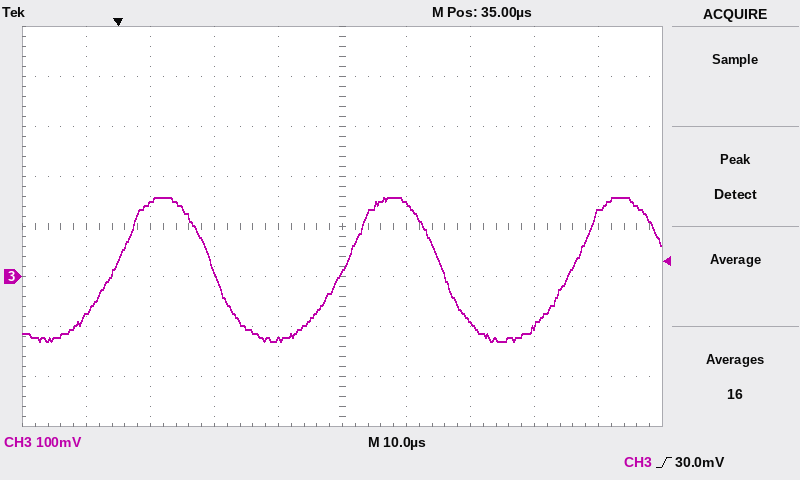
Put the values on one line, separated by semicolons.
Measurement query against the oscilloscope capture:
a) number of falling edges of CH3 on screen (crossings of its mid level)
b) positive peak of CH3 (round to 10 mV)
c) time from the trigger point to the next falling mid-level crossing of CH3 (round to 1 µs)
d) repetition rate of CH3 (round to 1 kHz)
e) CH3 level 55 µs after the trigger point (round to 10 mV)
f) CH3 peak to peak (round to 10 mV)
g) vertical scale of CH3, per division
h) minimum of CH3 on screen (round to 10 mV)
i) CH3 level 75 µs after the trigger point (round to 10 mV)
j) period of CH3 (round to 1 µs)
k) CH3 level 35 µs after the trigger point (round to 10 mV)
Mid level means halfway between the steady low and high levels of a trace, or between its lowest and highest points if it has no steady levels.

2; 160 mV; 15 µs; 28 kHz; -90 mV; 290 mV; 100 mV; -130 mV; 130 mV; 36 µs; 10 mV
